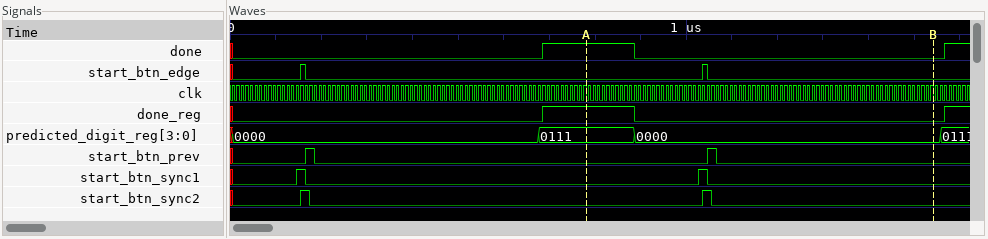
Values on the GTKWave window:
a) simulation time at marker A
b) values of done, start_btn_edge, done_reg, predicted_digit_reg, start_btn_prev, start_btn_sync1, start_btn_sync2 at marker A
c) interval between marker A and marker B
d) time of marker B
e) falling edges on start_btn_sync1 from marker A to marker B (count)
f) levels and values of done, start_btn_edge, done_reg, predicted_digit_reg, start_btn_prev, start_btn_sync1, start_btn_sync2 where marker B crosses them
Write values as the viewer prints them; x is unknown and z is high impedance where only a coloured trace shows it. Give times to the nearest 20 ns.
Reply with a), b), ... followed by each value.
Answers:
a) 780 ns
b) done=1, start_btn_edge=0, done_reg=1, predicted_digit_reg=0111, start_btn_prev=0, start_btn_sync1=0, start_btn_sync2=0
c) 760 ns
d) 1540 ns
e) 1
f) done=0, start_btn_edge=0, done_reg=0, predicted_digit_reg=0000, start_btn_prev=0, start_btn_sync1=0, start_btn_sync2=0
